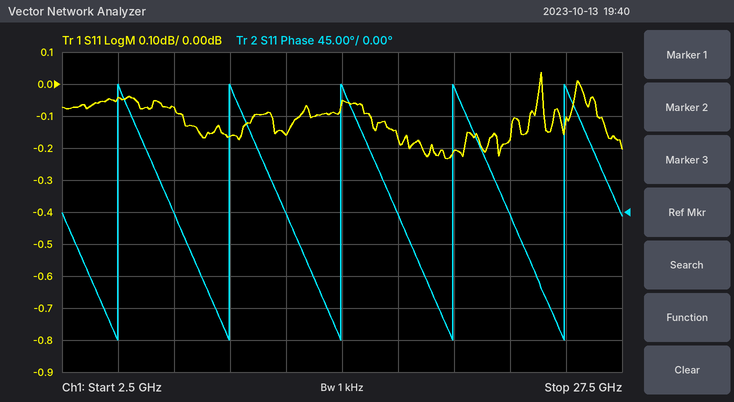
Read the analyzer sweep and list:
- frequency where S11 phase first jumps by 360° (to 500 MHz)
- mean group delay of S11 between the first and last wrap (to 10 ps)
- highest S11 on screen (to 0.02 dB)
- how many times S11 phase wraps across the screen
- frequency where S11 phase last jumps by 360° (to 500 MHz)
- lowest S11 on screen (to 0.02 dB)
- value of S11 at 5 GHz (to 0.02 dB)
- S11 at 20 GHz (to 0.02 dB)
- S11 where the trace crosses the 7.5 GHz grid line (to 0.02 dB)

5.0 GHz
200 ps
0.04 dB
5
25.0 GHz
-0.24 dB
-0.04 dB
-0.20 dB
-0.08 dB
